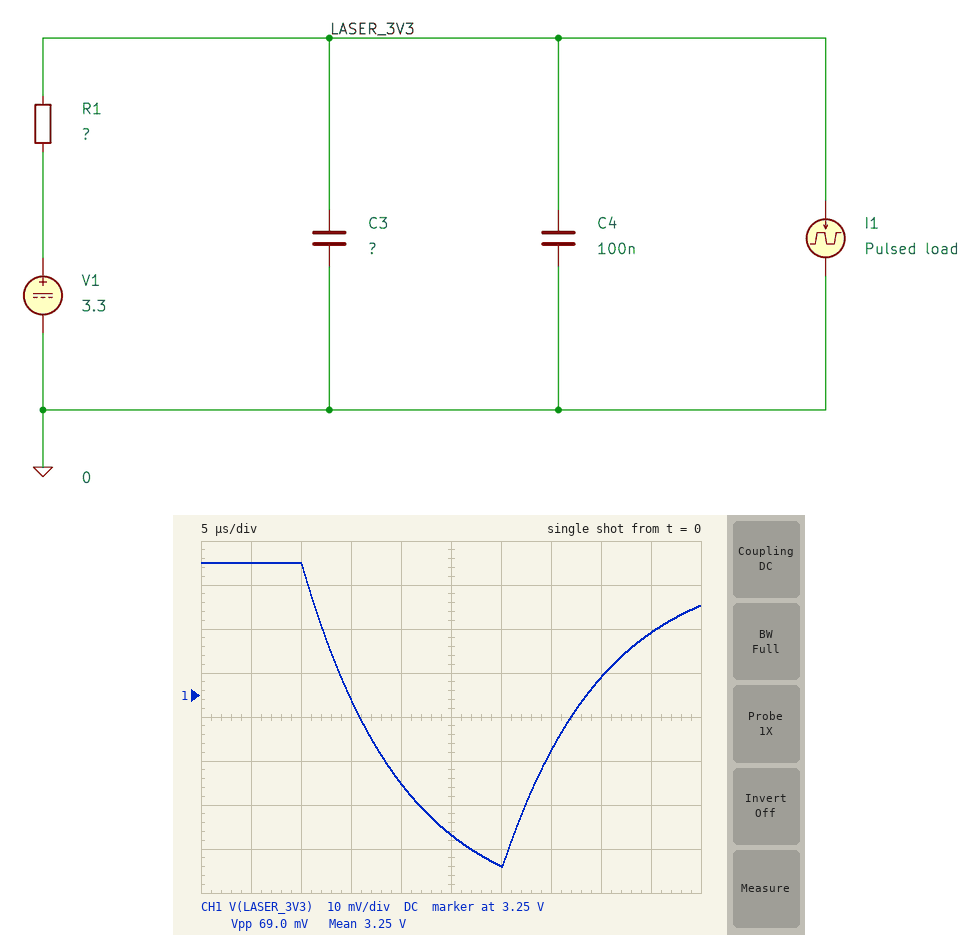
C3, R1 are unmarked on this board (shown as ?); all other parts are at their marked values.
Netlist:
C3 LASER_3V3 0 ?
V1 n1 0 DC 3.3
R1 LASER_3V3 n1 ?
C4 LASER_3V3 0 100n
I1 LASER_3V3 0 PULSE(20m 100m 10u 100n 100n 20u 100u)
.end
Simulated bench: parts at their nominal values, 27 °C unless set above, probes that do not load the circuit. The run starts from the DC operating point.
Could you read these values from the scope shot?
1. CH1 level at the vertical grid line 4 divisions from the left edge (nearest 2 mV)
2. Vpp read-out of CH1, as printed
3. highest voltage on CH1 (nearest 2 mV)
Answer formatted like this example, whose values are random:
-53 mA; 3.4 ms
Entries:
3.230 V; 69.0 mV; 3.280 V
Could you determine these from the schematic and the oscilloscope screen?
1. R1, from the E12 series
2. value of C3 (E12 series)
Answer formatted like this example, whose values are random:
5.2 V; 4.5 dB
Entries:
1 Ω; 10 µF
